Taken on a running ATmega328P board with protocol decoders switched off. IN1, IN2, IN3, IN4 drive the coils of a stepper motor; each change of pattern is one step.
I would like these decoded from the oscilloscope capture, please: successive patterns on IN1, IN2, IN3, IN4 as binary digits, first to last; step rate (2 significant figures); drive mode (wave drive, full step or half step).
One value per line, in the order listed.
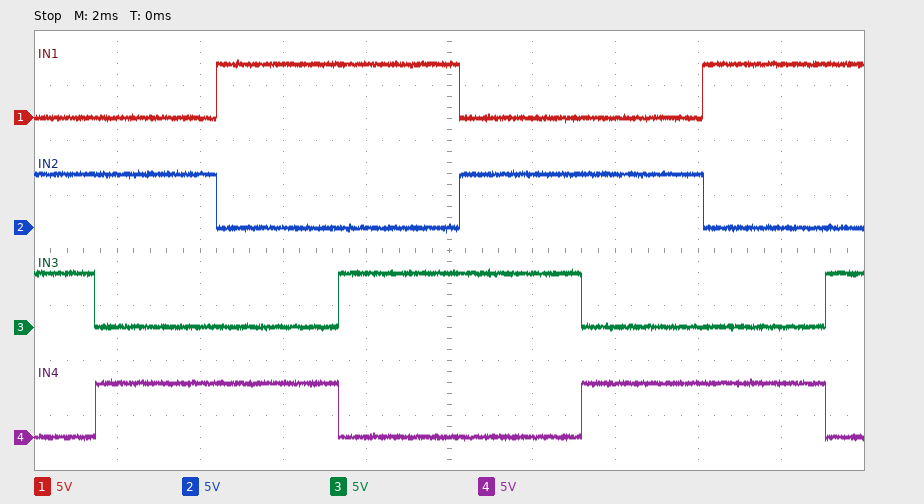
0110 0101 1001 1010 0110 0101 1001 1010
340 steps/s
full step
